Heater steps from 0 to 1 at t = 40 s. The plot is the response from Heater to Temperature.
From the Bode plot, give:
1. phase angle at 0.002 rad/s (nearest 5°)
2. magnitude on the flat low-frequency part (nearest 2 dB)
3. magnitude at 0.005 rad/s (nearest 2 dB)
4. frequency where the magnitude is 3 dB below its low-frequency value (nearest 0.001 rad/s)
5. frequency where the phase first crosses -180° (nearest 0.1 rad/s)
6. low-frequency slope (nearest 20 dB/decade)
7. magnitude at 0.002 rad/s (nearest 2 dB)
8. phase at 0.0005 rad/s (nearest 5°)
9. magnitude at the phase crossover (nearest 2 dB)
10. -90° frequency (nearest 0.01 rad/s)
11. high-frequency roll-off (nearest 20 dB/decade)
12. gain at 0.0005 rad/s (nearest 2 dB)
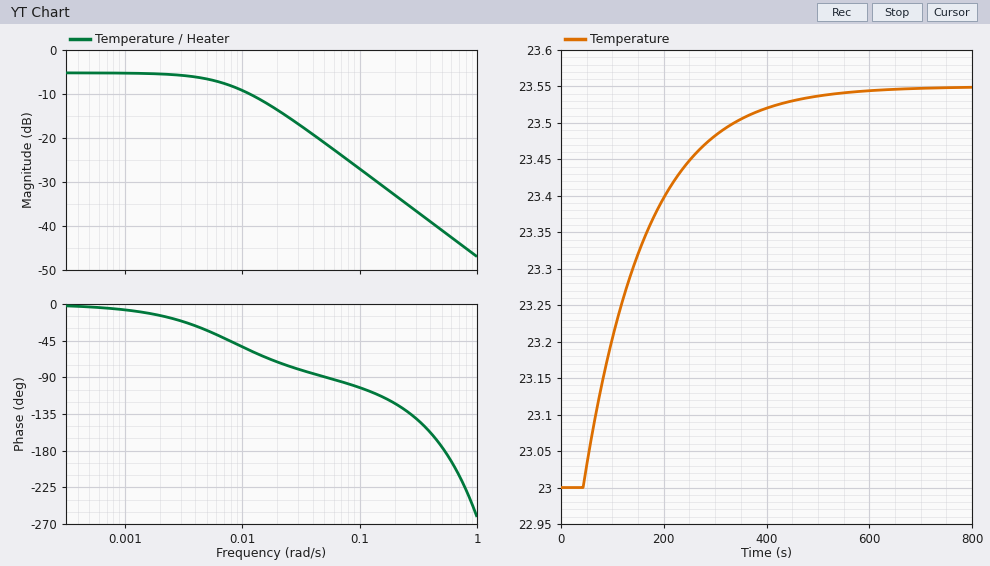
-15°
-6 dB
-6 dB
0.008 rad/s
0.5 rad/s
0 dB/decade
-6 dB
-5°
-42 dB
0.05 rad/s
-20 dB/decade
-6 dB
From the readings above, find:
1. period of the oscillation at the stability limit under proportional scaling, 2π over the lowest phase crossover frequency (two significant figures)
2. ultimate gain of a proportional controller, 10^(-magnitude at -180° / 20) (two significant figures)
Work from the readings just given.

13 s
130
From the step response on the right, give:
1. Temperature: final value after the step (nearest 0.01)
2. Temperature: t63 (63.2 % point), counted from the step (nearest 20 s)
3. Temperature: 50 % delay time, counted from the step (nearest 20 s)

23.55
120 s
80 s
